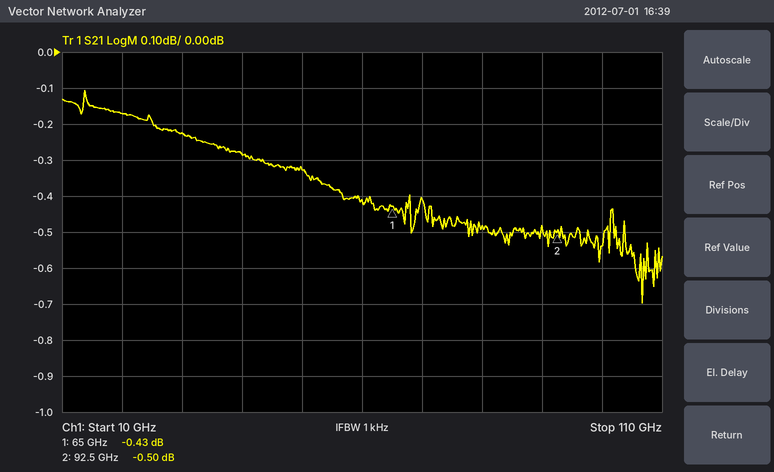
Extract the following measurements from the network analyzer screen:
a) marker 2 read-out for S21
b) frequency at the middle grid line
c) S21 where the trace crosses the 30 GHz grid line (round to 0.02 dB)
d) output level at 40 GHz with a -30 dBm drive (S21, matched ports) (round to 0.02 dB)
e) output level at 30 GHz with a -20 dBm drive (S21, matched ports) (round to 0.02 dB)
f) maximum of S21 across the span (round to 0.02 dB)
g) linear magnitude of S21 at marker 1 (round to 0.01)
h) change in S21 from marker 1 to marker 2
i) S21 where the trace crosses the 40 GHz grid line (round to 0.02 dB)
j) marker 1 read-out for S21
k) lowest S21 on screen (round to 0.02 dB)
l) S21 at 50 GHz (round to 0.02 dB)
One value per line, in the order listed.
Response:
-0.50 dB
60 GHz
-0.22 dB
-30.28 dBm
-20.22 dBm
-0.10 dB
0.95
-0.07 dB
-0.28 dB
-0.43 dB
-0.70 dB
-0.32 dB
